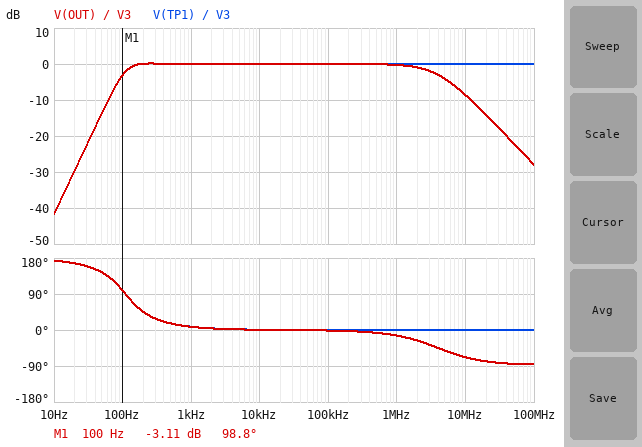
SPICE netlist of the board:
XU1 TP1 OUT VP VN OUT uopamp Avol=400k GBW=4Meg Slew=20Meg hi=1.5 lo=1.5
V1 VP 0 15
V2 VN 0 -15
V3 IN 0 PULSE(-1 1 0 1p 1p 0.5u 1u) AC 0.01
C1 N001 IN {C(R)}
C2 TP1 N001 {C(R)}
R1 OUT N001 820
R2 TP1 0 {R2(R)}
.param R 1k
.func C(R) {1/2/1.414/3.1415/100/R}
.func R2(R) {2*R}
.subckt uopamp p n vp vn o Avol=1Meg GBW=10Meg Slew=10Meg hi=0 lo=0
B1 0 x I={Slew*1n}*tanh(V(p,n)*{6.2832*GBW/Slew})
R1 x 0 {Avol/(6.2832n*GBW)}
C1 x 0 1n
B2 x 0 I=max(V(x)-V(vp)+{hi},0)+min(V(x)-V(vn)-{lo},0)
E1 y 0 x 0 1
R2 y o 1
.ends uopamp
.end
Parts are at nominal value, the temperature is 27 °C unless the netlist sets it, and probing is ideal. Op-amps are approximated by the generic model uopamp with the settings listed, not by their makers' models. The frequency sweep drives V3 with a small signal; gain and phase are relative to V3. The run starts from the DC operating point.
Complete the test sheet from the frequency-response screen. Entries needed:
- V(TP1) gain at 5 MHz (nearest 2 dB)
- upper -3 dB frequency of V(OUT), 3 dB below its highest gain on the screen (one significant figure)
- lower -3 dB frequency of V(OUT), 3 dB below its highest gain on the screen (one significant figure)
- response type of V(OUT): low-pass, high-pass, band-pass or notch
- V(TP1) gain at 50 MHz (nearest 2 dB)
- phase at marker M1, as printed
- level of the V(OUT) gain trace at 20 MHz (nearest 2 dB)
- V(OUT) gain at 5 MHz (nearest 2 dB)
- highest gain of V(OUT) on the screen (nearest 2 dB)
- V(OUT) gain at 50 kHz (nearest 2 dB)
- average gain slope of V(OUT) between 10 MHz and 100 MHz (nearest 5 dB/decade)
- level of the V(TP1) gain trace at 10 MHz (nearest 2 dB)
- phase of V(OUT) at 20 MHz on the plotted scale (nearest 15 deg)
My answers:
0 dB
4 MHz
100 Hz
band-pass
0 dB
98.8 deg
-14 dB
-4 dB
0 dB
0 dB
-20 dB/decade
0 dB
-75 deg
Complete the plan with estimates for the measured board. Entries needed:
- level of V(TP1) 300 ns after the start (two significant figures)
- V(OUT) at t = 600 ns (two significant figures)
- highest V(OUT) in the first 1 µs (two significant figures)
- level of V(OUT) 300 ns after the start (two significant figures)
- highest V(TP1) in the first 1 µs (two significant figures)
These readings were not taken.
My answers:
2.0 V
380 mV
2.0 V
2.0 V
2.0 V
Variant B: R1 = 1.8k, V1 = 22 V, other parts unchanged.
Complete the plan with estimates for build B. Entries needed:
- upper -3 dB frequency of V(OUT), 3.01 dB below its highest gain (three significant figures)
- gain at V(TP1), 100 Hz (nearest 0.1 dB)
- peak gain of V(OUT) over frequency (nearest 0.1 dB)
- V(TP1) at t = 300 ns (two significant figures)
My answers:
4.00 MHz
-3.4 dB
0 dB
2.0 V
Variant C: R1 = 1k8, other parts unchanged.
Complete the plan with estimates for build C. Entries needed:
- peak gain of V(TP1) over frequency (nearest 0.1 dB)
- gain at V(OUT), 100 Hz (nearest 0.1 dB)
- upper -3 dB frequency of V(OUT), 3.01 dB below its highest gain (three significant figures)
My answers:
0 dB
-3.4 dB
4.00 MHz
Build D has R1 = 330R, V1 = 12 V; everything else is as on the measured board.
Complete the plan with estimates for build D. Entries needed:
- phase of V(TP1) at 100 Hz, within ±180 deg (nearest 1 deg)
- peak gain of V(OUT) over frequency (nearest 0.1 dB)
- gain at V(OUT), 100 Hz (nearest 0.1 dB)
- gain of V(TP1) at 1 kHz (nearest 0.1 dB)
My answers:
145 deg
2.6 dB
-7.9 dB
0.2 dB
